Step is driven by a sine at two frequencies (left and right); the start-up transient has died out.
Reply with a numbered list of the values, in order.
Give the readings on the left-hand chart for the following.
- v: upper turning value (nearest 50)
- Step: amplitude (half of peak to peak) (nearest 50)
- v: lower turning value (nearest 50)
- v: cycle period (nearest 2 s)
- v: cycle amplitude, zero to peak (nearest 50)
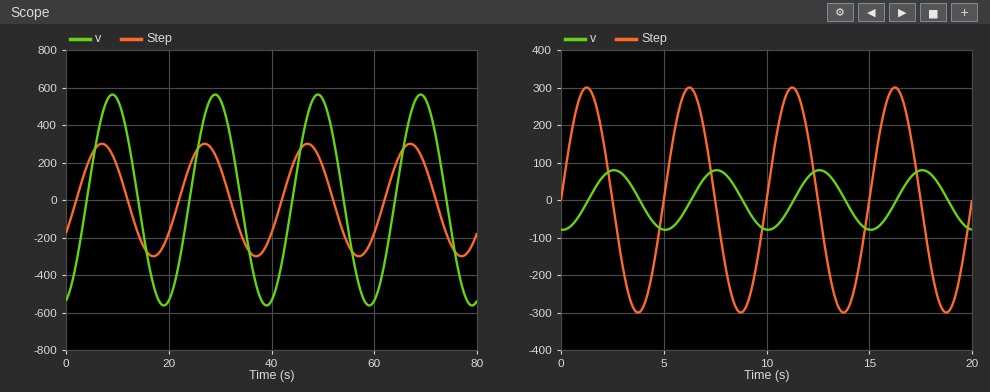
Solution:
1. 550
2. 300
3. -550
4. 20 s
5. 550
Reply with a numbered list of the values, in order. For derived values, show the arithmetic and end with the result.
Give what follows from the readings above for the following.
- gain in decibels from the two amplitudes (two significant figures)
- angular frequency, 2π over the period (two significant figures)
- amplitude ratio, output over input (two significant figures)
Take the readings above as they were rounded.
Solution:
1. 20 log10(550 / 300) = 5.3 dB
2. 2π / 20 = 0.31 rad/s
3. 550 / 300 = 1.8
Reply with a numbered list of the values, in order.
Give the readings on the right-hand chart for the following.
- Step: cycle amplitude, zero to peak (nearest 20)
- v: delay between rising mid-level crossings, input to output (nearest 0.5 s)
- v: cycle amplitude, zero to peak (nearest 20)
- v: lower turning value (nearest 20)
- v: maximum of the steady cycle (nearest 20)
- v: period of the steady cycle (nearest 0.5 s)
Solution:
1. 300
2. 1.5 s
3. 80
4. -80
5. 80
6. 5.0 s
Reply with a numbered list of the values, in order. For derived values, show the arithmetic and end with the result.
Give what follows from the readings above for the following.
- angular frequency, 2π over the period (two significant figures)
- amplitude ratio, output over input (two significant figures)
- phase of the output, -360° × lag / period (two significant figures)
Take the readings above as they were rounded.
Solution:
1. 2π / 5 = 1.3 rad/s
2. 80 / 300 = 0.27
3. -360 × 1.5 / 5 = -110°
